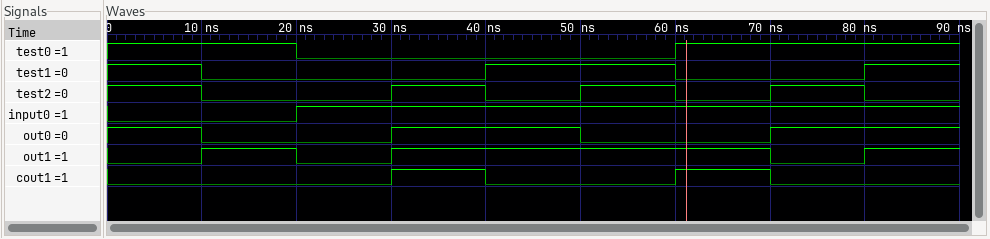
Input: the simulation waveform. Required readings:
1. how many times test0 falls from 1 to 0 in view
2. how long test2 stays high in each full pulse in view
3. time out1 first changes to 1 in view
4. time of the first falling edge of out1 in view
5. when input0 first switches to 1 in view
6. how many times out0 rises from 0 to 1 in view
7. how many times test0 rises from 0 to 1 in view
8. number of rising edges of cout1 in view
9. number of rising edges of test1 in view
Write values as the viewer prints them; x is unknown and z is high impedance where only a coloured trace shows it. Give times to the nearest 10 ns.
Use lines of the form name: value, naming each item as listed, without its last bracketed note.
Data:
how many times test0 falls from 1 to 0 in view: 1
how long test2 stays high in each full pulse in view: 10 ns, 10 ns, 10 ns
time out1 first changes to 1 in view: 10 ns
time of the first falling edge of out1 in view: 20 ns
when input0 first switches to 1 in view: 20 ns
how many times out0 rises from 0 to 1 in view: 2
how many times test0 rises from 0 to 1 in view: 1
number of rising edges of cout1 in view: 2
number of rising edges of test1 in view: 2
